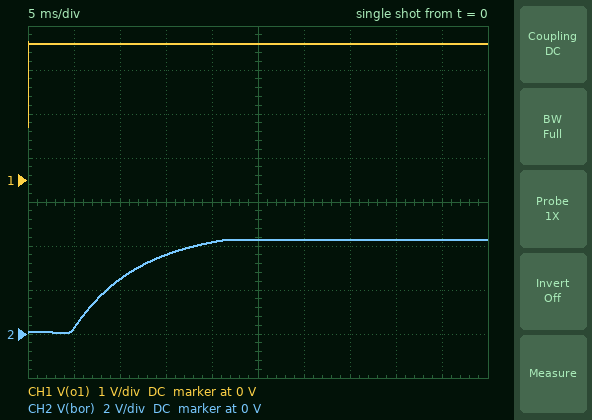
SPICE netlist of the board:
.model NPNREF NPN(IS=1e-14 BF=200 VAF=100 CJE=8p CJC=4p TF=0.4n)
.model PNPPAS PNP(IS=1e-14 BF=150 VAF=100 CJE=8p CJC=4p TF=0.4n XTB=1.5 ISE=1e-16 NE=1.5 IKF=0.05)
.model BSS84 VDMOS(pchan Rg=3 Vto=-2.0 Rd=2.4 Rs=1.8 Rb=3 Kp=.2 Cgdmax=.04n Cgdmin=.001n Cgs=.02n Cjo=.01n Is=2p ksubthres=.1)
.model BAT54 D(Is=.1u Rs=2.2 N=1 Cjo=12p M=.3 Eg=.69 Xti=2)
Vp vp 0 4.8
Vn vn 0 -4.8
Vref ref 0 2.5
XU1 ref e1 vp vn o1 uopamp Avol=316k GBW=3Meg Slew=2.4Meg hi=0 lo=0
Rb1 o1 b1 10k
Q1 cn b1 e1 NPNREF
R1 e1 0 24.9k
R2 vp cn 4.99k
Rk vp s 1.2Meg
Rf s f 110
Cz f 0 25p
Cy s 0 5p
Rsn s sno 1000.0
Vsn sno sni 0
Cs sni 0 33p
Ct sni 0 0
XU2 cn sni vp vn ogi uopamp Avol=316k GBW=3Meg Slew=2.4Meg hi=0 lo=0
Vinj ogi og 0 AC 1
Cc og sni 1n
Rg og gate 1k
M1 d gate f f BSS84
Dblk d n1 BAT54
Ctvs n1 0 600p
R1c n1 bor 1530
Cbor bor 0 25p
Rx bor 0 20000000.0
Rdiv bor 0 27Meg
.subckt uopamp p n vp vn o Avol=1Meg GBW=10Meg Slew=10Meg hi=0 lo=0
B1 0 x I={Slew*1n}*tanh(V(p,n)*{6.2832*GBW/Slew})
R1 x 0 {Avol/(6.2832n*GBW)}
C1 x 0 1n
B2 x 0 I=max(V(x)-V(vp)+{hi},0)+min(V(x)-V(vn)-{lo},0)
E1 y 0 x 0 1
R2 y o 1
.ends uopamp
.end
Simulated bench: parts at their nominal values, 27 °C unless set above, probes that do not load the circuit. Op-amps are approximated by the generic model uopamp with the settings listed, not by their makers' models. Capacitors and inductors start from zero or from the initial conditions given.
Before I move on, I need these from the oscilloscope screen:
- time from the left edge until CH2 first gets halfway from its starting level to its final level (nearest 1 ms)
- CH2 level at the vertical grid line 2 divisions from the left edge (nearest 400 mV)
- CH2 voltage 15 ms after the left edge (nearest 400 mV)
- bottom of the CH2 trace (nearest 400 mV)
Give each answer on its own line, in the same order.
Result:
9 ms
2.4 V
3.6 V
0 V
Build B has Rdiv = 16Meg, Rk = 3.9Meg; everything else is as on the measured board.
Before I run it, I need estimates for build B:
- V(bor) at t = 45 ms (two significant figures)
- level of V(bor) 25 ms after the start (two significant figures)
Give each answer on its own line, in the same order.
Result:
1.1 V
950 mV
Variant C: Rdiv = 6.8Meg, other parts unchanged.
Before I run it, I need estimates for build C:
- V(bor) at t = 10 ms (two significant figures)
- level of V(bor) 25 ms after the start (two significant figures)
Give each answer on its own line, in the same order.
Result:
1.7 V
2.1 V
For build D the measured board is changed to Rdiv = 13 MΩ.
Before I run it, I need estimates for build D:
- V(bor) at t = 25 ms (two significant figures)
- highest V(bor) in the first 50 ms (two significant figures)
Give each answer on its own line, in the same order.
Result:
3.2 V
3.3 V
